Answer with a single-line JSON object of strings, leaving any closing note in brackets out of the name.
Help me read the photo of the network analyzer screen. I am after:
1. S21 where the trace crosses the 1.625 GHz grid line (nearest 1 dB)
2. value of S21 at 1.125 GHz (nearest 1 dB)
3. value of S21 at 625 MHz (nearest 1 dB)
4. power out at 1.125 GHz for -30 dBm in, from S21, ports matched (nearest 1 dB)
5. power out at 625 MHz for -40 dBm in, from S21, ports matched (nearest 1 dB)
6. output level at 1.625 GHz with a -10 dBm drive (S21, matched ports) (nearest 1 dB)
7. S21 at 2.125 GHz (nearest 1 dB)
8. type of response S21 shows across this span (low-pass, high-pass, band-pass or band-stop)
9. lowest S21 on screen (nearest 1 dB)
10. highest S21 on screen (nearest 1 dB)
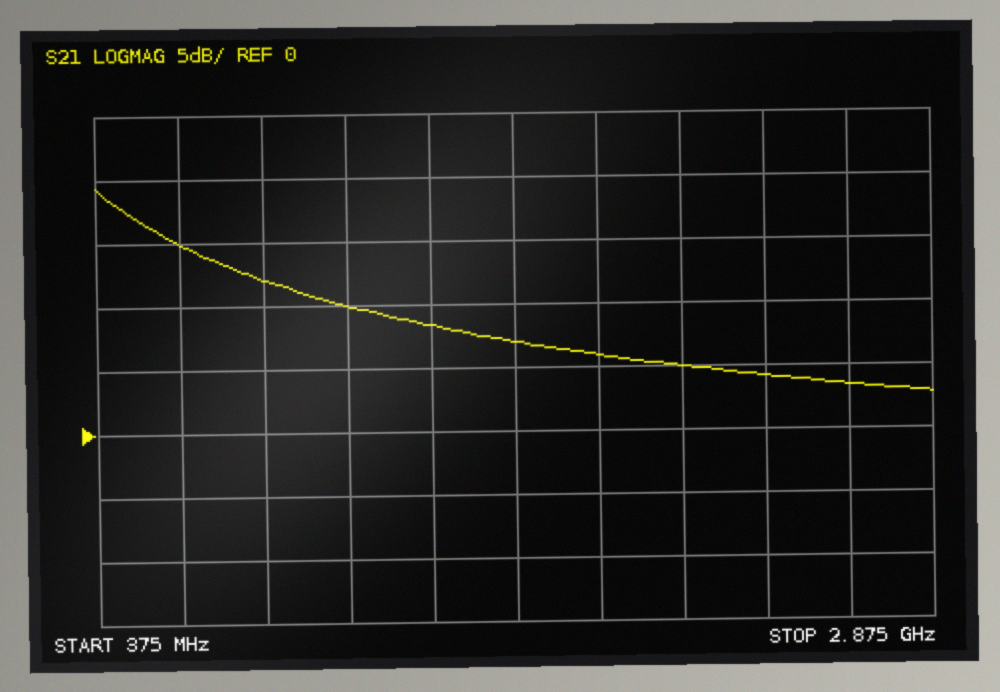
{"S21 where the trace crosses the 1.625 GHz grid line": "7 dB", "value of S21 at 1.125 GHz": "10 dB", "value of S21 at 625 MHz": "15 dB", "power out at 1.125 GHz for -30 dBm in, from S21, ports matched": "-20 dBm", "power out at 625 MHz for -40 dBm in, from S21, ports matched": "-25 dBm", "output level at 1.625 GHz with a -10 dBm drive (S21, matched ports)": "-3 dBm", "S21 at 2.125 GHz": "5 dB", "type of response S21 shows across this span": "low-pass", "lowest S21 on screen": "3 dB", "highest S21 on screen": "19 dB"}
